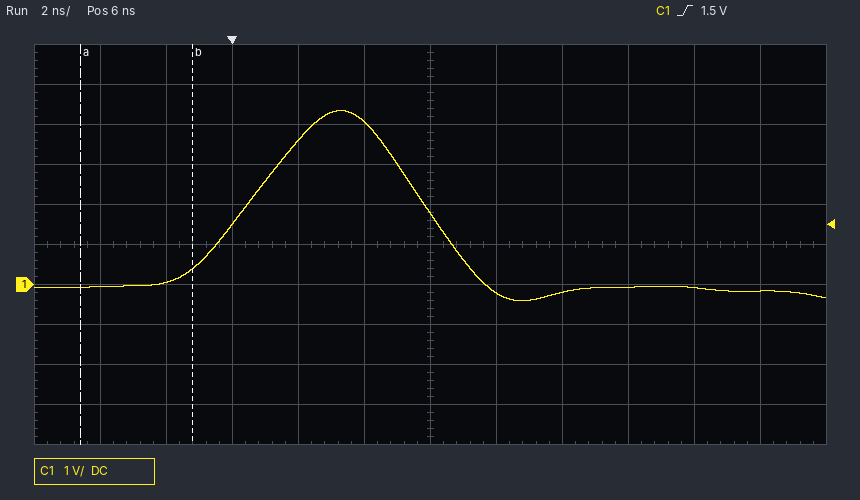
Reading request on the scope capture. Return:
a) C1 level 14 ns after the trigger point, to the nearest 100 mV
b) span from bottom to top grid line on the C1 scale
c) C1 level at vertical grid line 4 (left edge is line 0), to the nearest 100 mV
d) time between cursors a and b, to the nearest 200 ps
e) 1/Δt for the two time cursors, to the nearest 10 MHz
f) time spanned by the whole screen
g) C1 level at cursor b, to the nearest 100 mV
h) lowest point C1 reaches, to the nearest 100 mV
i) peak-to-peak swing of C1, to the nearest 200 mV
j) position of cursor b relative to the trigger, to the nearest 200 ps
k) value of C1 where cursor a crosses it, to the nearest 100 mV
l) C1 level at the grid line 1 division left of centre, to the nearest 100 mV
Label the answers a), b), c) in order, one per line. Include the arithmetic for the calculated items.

a) -100 mV
b) 10 V
c) 3.6 V
d) 3.4 ns
e) 1 / 3.4 ns ≈ 290 MHz
f) 24 ns
g) 400 mV
h) -400 mV
i) 4.8 V
j) -1.2 ns
k) -100 mV
l) 4.1 V
